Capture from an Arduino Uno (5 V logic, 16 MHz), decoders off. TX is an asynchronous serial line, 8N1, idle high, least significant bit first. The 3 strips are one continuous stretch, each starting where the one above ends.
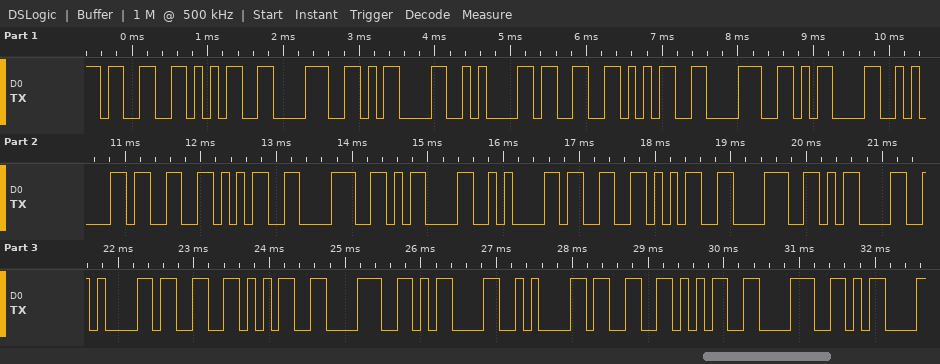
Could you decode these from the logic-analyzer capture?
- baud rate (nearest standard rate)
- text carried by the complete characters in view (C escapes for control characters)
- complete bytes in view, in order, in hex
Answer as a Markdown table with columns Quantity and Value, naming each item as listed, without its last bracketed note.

| Quantity | Value |
|---|---|
| baud rate | 9600 baud |
| text carried by the complete characters in view | "358\r\n358\r\n358\r\n358\r\n358\r\n358\r" |
| complete bytes in view, in order, in hex | 0x33 0x35 0x38 0x0D 0x0A 0x33 0x35 0x38 0x0D 0x0A 0x33 0x35 0x38 0x0D 0x0A 0x33 0x35 0x38 0x0D 0x0A 0x33 0x35 0x38 0x0D 0x0A 0x33 0x35 0x38 0x0D |
